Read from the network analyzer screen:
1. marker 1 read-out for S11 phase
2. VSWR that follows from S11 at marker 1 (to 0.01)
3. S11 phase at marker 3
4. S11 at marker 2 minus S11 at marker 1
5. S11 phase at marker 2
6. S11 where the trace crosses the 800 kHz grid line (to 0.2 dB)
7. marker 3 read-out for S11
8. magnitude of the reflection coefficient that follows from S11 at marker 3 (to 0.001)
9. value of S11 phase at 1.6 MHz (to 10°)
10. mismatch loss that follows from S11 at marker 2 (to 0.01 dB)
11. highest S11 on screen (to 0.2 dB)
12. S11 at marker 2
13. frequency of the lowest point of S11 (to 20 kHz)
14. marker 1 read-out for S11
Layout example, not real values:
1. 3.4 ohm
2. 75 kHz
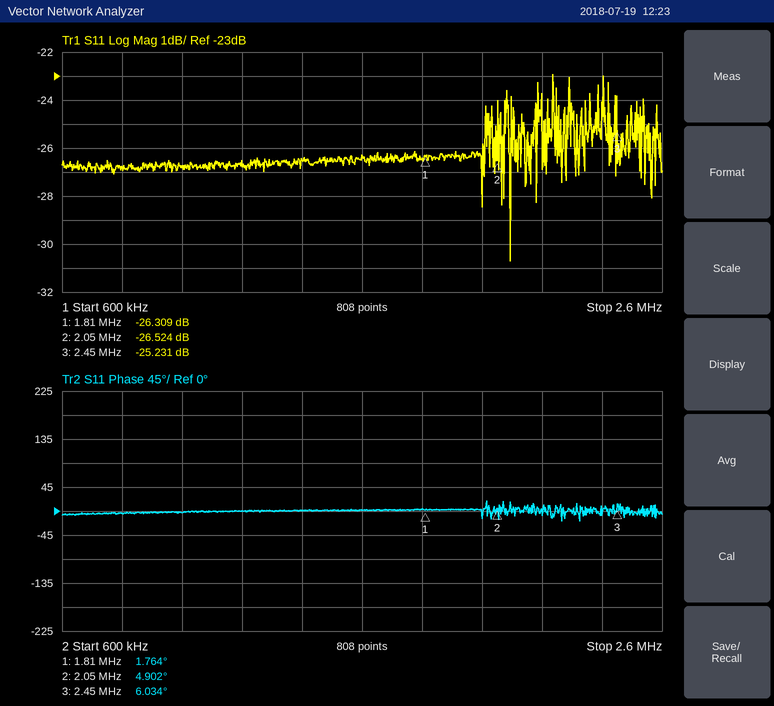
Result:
1. 1.764°
2. 1.10
3. 6.034°
4. -0.215 dB
5. 4.902°
6. -26.8 dB
7. -25.231 dB
8. 0.055
9. 0°
10. 0.01 dB
11. -23.0 dB
12. -26.524 dB
13. 2.10 MHz
14. -26.309 dB
